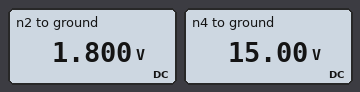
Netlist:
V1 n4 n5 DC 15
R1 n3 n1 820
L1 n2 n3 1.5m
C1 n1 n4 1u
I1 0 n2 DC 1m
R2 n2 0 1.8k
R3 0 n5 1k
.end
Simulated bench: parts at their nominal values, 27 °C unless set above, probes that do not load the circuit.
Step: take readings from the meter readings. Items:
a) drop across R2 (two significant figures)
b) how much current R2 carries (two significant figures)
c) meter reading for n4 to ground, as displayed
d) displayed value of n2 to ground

1.8 V
1.0 mA
15.00 V
1.800 V
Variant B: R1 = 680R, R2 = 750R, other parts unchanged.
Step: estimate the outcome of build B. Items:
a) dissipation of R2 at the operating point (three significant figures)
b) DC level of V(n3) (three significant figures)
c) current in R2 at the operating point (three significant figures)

750 µW
750 mV
1.00 mA
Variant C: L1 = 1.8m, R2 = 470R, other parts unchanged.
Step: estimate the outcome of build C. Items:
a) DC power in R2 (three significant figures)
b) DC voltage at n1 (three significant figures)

470 µW
470 mV
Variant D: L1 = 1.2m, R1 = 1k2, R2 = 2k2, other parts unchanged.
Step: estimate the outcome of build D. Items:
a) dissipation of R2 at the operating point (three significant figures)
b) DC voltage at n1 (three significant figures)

2.20 mW
2.20 V
